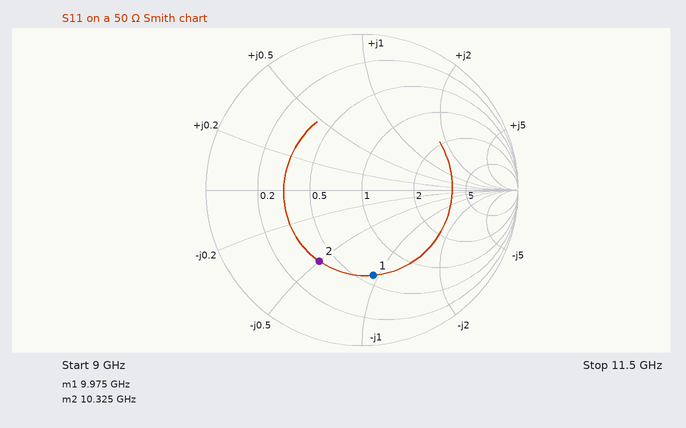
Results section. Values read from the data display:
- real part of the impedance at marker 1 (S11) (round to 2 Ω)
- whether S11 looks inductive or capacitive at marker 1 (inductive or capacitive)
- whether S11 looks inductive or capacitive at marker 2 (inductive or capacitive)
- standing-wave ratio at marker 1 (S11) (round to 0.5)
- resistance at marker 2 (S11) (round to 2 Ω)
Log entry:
30 Ω
capacitive
capacitive
3.5
20 Ω
